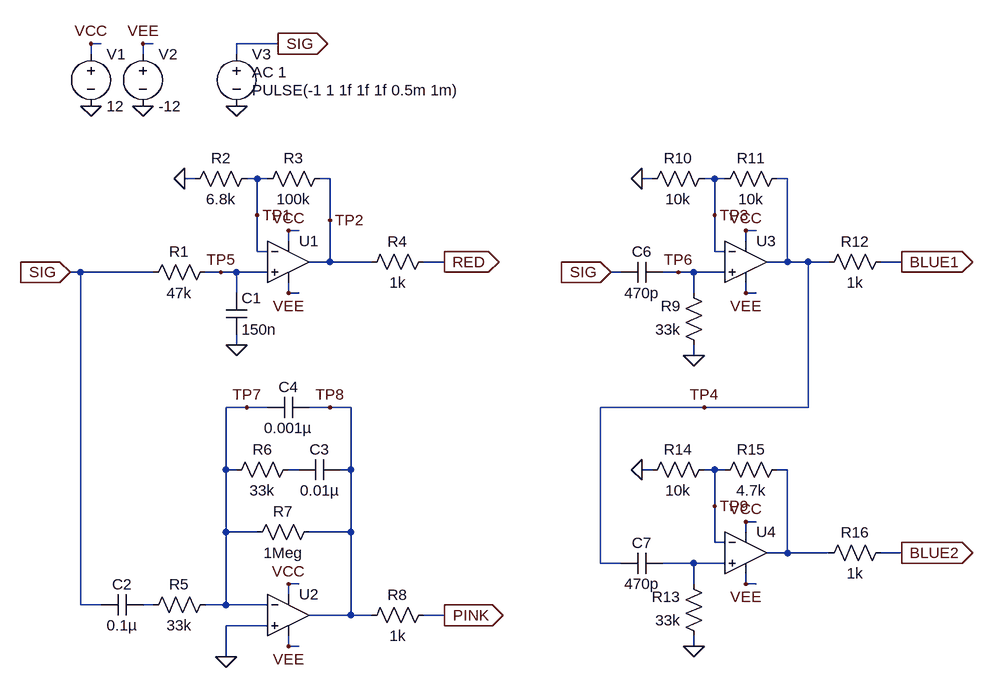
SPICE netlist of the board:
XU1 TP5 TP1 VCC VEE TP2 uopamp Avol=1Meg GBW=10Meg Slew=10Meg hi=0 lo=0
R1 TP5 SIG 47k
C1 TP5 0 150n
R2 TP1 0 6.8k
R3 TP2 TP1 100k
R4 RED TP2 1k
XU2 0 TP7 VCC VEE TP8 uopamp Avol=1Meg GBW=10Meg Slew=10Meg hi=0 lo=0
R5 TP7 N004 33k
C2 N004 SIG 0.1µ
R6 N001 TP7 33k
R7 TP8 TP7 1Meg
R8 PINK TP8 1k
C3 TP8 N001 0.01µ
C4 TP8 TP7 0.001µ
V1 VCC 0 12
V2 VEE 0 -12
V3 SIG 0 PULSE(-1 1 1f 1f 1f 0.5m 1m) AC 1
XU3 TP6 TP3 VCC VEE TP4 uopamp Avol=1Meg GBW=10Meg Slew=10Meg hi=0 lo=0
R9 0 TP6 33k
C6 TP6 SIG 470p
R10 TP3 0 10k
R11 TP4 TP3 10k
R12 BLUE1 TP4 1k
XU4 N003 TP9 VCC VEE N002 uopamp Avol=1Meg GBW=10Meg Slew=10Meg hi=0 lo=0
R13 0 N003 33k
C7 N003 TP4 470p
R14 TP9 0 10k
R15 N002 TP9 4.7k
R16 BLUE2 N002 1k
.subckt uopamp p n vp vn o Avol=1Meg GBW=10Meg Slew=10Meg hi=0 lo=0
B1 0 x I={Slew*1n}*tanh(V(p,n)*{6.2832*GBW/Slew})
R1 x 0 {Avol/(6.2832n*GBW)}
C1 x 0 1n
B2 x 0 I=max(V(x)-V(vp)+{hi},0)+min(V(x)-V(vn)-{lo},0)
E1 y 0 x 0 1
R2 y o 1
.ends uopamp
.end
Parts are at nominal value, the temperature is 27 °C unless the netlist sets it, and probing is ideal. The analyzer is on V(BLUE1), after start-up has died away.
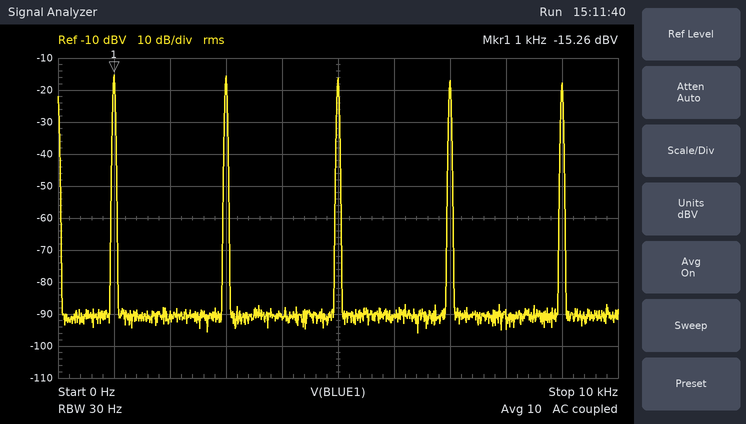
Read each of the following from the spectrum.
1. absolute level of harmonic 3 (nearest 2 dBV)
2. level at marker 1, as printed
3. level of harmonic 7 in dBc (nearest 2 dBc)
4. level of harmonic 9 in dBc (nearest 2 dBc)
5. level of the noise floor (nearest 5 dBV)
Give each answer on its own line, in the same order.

-16 dBV
-15.26 dBV
-2 dBc
-2 dBc
-90 dBV
